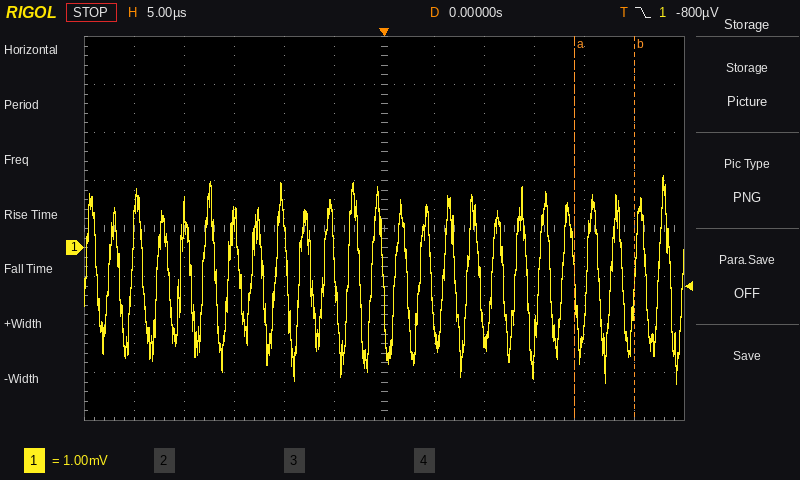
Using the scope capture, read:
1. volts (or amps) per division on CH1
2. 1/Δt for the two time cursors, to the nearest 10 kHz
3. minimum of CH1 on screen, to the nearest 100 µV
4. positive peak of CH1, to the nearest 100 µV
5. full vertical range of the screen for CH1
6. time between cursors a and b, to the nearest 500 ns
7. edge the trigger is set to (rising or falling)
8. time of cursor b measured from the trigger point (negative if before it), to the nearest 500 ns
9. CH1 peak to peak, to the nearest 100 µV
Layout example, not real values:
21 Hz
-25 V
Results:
1 mV
170 kHz
-2.8 mV
1.5 mV
8 mV
6.0 µs
falling
+25.0 µs
4.3 mV
